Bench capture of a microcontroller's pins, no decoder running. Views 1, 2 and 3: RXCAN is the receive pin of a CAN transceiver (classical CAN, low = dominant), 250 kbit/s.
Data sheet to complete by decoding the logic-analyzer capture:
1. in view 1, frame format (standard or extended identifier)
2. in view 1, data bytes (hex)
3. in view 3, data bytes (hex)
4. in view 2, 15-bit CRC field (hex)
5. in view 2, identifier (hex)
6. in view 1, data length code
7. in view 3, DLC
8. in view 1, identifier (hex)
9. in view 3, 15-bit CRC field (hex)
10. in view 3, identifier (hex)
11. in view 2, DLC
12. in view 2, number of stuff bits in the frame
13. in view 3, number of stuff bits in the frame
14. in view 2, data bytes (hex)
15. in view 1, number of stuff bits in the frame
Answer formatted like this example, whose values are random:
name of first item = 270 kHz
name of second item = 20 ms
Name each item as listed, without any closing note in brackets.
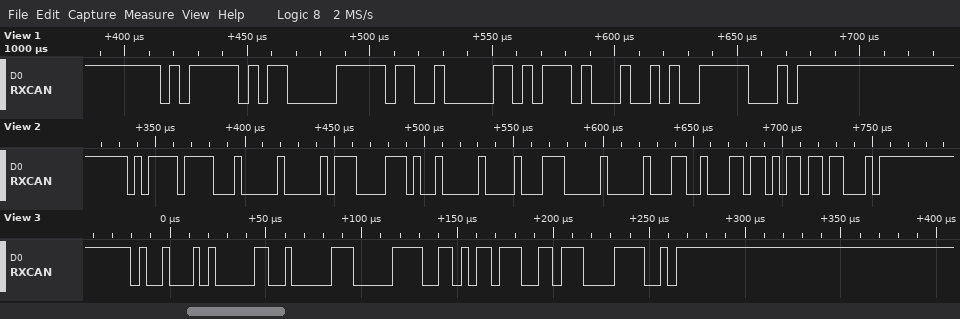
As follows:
in view 1, frame format = standard
in view 1, data bytes = F2 0A E8
in view 3, data bytes = 83 07 35 B9
in view 2, 15-bit CRC field = 0x56D8
in view 2, identifier = 0x5EF
in view 1, data length code = 3
in view 3, DLC = 4
in view 1, identifier = 0x5FB
in view 3, 15-bit CRC field = 0x5C3C
in view 3, identifier = 0x48A
in view 2, DLC = 8
in view 2, number of stuff bits in the frame = 5
in view 3, number of stuff bits in the frame = 3
in view 2, data bytes = 00 E1 D2 00 8E 00 0C 8D
in view 1, number of stuff bits in the frame = 5
